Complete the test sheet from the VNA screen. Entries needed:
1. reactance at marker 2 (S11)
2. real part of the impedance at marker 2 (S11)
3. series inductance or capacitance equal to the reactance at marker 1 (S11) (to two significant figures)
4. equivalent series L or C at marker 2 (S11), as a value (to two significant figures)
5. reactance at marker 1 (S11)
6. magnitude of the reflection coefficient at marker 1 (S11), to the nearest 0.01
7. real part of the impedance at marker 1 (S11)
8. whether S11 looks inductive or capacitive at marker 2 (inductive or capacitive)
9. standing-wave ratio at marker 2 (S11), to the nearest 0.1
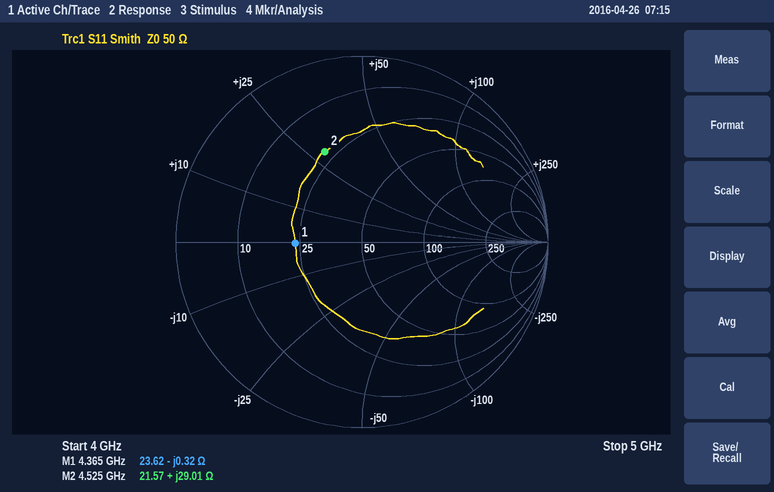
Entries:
+29.01 Ω
21.57 Ω
110 pF
1.0 nH
-0.32 Ω
0.36
23.62 Ω
inductive
3.2
